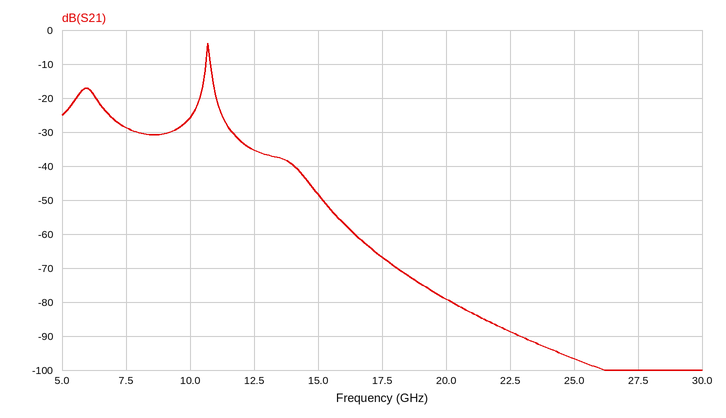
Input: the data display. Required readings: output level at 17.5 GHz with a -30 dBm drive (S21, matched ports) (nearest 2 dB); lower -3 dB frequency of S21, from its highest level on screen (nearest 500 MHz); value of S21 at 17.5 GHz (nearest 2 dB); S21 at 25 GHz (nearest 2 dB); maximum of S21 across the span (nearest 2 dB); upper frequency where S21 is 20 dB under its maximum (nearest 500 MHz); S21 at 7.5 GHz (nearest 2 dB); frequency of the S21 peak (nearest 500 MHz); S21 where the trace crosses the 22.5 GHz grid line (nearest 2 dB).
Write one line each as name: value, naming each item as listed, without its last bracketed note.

output level at 17.5 GHz with a -30 dBm drive (S21, matched ports): -96 dBm
lower -3 dB frequency of S21, from its highest level on screen: 10.5 GHz
value of S21 at 17.5 GHz: -66 dB
S21 at 25 GHz: -96 dB
maximum of S21 across the span: -4 dB
upper frequency where S21 is 20 dB under its maximum: 11.0 GHz
S21 at 7.5 GHz: -28 dB
frequency of the S21 peak: 10.5 GHz
S21 where the trace crosses the 22.5 GHz grid line: -88 dB
